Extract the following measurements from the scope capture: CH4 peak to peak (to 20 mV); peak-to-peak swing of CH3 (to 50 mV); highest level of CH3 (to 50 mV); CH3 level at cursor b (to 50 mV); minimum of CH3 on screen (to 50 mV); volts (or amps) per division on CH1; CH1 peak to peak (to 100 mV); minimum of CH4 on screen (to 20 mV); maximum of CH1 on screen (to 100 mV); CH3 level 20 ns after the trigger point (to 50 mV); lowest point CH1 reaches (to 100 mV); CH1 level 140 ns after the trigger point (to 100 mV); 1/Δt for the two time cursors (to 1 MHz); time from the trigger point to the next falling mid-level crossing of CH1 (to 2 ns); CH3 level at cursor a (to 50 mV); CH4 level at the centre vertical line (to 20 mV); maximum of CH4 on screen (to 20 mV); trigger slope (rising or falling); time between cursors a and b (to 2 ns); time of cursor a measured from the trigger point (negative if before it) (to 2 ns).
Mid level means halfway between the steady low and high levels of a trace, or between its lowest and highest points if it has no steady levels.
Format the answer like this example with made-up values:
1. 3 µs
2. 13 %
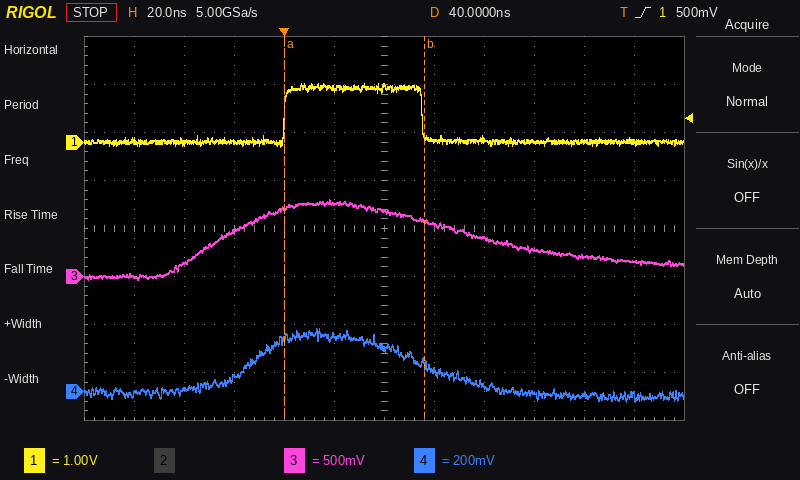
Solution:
1. 300 mV
2. 850 mV
3. 800 mV
4. 600 mV
5. -50 mV
6. 1 V
7. 1.3 V
8. -40 mV
9. 1.2 V
10. 750 mV
11. -100 mV
12. 0.0 V
13. 18 MHz
14. 56 ns
15. 700 mV
16. 180 mV
17. 260 mV
18. rising
19. 56 ns
20. 0 ns
